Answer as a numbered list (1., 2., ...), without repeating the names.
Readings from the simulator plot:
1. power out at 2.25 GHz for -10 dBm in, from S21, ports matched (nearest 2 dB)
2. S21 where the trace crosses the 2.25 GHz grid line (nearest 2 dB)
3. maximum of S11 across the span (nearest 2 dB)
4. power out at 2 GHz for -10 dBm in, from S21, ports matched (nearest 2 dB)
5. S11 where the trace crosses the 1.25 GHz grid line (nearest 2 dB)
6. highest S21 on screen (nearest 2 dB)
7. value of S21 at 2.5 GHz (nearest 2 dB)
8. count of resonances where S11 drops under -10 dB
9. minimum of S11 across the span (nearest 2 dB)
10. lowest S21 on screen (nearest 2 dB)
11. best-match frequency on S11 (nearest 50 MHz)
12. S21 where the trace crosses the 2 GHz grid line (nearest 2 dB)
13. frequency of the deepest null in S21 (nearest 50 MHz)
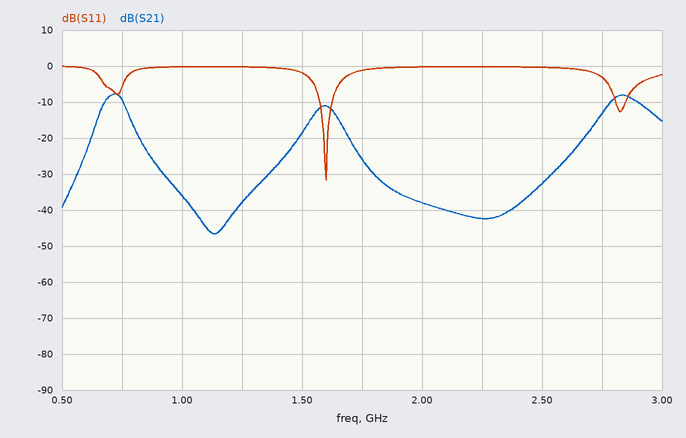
1. -52 dBm
2. -42 dB
3. 0 dB
4. -48 dBm
5. 0 dB
6. -8 dB
7. -32 dB
8. 2
9. -32 dB
10. -46 dB
11. 1.60 GHz
12. -38 dB
13. 1.15 GHz
